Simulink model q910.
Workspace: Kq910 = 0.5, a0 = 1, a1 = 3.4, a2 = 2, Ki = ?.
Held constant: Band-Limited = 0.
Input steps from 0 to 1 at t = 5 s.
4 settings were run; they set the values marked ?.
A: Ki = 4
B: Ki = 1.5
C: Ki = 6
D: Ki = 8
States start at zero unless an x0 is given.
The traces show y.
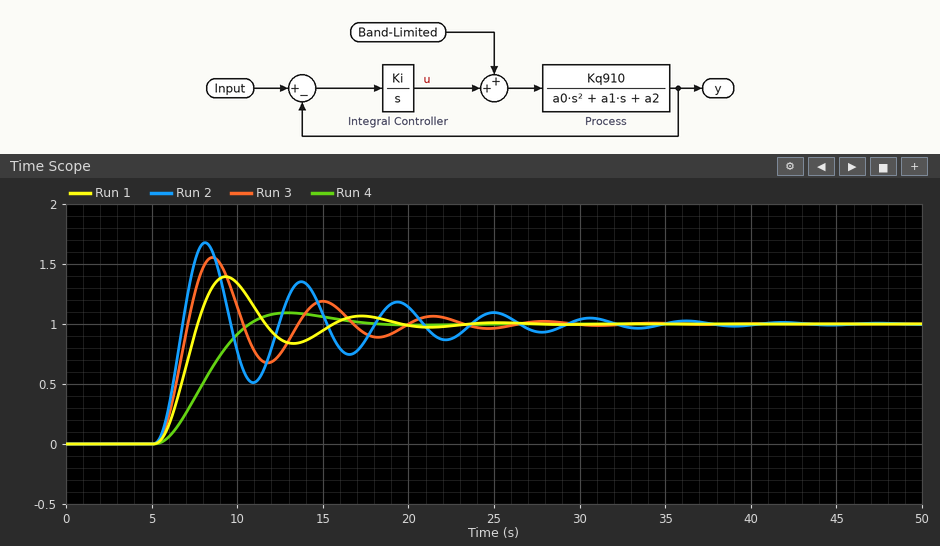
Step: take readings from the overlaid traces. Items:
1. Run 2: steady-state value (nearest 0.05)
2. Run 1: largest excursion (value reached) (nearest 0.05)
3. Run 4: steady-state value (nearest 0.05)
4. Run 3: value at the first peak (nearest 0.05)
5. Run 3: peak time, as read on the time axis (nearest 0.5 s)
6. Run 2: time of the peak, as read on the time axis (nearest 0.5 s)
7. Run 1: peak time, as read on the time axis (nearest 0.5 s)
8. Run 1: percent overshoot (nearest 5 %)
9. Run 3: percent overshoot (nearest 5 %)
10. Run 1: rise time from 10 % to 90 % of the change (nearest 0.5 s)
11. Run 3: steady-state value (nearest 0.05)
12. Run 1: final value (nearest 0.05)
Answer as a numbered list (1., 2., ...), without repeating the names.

1. 1.00
2. 1.40
3. 1.00
4. 1.55
5. 8.5 s
6. 8.0 s
7. 9.5 s
8. 40 %
9. 55 %
10. 1.5 s
11. 1.00
12. 1.00
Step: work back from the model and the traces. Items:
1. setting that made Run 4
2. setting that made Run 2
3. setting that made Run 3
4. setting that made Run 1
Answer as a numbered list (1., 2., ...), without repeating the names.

1. B
2. D
3. C
4. A
